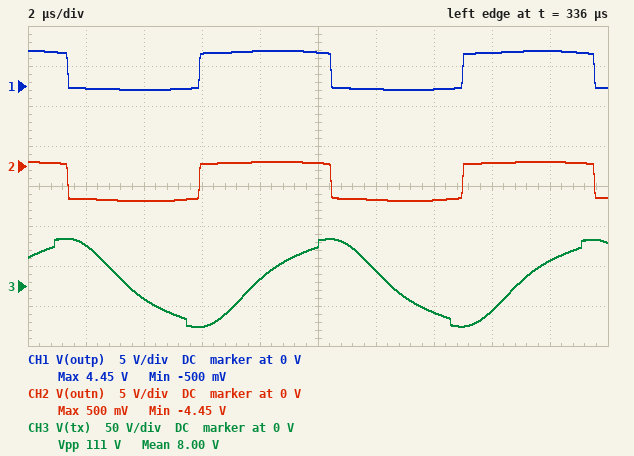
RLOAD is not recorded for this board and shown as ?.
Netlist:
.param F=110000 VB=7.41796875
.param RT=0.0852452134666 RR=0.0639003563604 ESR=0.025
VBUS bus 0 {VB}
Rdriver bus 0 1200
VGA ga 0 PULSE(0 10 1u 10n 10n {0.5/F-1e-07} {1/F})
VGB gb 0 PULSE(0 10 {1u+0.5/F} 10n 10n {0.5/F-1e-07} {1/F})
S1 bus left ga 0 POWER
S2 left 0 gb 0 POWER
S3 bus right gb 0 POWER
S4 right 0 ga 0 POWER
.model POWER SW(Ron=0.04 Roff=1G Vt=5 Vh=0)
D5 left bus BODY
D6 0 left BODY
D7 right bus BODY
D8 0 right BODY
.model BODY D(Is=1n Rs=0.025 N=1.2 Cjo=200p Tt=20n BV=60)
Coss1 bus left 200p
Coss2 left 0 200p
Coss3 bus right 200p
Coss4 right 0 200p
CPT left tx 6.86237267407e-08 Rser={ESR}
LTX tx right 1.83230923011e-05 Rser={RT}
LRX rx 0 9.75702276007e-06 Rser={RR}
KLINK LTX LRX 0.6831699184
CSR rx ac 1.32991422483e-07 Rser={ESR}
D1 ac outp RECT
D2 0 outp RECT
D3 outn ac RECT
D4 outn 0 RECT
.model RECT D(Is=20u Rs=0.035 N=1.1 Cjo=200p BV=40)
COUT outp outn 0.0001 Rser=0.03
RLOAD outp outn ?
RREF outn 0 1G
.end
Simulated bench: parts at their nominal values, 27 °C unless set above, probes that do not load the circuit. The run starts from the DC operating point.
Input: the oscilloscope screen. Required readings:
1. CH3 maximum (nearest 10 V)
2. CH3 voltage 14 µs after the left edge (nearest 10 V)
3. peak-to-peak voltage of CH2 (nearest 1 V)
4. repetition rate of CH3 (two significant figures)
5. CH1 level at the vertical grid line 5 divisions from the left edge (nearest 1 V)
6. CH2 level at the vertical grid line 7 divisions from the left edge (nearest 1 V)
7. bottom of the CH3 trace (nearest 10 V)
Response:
60 V
-30 V
5 V
110 kHz
4 V
-4 V
-50 V
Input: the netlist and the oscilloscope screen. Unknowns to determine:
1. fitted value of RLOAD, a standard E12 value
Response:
1.5 Ω
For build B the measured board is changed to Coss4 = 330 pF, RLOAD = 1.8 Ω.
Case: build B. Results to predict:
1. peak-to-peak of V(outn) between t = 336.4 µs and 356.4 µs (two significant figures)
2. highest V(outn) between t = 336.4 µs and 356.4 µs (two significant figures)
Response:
5.1 V
470 mV
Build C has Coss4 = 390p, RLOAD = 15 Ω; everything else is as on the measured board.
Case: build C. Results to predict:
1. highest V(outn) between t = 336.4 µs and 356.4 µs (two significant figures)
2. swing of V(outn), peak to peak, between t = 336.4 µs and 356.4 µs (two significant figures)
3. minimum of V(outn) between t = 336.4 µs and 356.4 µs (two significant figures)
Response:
330 mV
6.8 V
-6.5 V
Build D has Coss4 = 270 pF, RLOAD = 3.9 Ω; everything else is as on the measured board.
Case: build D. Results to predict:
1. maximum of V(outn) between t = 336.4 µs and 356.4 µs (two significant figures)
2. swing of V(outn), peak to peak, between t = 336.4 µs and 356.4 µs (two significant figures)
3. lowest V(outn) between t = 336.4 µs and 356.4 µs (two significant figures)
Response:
390 mV
5.9 V
-5.5 V
